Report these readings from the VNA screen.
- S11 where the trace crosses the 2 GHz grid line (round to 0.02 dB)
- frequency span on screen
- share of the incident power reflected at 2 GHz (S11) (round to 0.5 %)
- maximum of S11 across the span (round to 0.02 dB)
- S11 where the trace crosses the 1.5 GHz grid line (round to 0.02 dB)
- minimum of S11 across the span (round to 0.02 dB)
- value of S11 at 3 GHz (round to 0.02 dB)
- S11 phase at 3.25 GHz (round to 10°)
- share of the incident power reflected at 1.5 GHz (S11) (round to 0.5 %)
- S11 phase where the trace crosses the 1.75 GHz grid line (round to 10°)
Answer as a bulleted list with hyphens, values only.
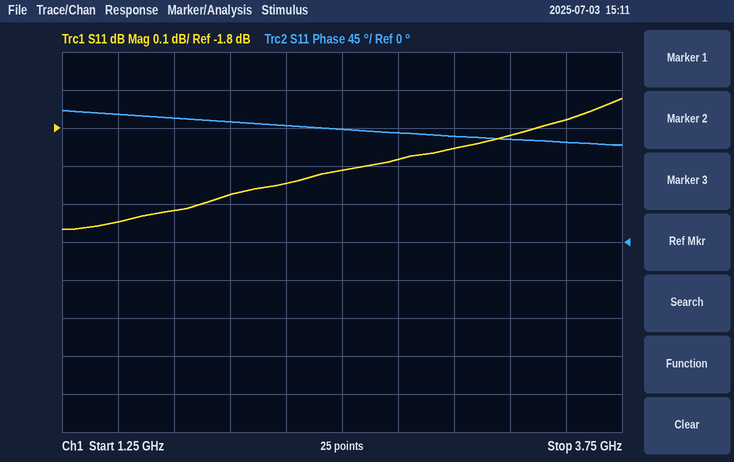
- -1.98 dB
- 2.5 GHz
- 63.5 %
- -1.72 dB
- -2.04 dB
- -2.06 dB
- -1.86 dB
- 120°
- 62.5 %
- 150°
